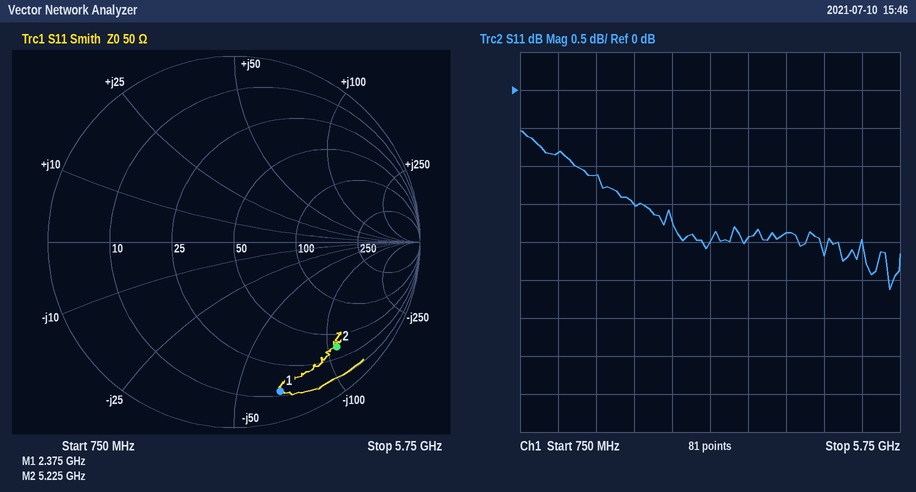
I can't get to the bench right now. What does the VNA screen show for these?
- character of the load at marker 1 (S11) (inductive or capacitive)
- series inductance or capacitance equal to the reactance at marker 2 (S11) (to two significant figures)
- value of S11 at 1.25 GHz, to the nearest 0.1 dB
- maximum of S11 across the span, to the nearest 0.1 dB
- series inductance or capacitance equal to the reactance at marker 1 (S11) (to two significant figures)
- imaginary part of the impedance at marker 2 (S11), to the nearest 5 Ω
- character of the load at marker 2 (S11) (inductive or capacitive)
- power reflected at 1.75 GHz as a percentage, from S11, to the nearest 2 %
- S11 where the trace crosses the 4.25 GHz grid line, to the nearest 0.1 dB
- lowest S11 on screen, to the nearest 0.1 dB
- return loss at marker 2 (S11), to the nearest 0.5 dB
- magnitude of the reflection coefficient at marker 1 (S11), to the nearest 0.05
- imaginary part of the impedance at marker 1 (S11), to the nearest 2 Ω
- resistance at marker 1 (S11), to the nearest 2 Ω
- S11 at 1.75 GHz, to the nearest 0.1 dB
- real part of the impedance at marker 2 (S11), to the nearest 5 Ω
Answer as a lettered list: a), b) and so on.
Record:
a) capacitive
b) 280 fF
c) -0.8 dB
d) -0.5 dB
e) 1.0 pF
f) -110 Ω
g) capacitive
h) 78 %
i) -1.9 dB
j) -2.6 dB
k) 2.0 dB
l) 0.85
m) -66 Ω
n) 12 Ω
o) -1.1 dB
p) 35 Ω
